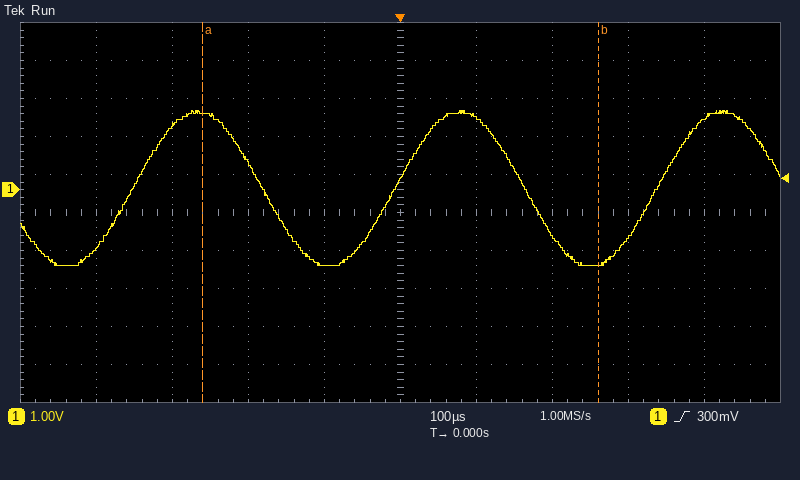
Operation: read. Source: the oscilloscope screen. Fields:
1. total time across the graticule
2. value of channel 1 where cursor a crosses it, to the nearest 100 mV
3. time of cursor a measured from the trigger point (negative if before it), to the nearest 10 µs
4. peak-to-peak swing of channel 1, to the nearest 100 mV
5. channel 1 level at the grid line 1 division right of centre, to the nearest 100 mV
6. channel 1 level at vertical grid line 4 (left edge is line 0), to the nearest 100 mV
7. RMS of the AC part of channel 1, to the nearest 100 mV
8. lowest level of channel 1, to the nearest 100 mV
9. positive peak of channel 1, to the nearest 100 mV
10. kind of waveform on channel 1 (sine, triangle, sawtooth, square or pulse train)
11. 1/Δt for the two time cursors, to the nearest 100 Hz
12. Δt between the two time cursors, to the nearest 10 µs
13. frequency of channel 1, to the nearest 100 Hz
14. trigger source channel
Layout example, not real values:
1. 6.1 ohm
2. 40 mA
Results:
1. 1 ms
2. 2.0 V
3. -260 µs
4. 4.1 V
5. 1.9 V
6. -2.0 V
7. 1.4 V
8. -2.0 V
9. 2.1 V
10. sine
11. 1.9 kHz
12. 520 µs
13. 2.9 kHz
14. channel 1
